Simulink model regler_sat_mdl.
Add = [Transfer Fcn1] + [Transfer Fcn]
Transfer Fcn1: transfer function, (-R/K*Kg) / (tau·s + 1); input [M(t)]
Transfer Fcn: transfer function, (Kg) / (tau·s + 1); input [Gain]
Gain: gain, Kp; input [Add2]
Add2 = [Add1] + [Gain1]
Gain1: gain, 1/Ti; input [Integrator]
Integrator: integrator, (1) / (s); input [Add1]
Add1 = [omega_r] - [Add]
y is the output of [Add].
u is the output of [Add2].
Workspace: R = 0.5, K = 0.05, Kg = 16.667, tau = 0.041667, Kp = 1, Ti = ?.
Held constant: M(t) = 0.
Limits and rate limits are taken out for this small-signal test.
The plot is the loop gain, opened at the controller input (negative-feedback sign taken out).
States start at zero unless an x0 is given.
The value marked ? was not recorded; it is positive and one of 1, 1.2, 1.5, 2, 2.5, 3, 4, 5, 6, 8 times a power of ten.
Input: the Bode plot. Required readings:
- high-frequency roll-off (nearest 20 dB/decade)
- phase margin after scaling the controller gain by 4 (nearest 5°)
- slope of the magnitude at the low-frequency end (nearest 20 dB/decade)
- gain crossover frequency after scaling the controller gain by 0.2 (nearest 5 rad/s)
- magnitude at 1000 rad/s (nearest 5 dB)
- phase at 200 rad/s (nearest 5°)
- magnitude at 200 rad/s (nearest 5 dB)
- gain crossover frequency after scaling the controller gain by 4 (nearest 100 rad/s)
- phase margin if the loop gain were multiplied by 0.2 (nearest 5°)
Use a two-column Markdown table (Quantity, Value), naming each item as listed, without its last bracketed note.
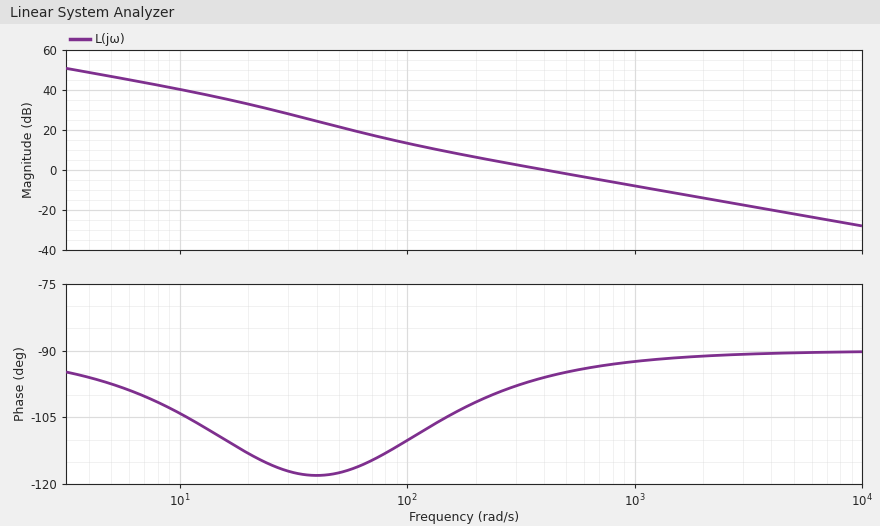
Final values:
| Quantity | Value |
|---|---|
| high-frequency roll-off | -20 dB/decade |
| phase margin after scaling the controller gain by 4 | 90° |
| slope of the magnitude at the low-frequency end | -20 dB/decade |
| gain crossover frequency after scaling the controller gain by 0.2 | 95 rad/s |
| magnitude at 1000 rad/s | -10 dB |
| phase at 200 rad/s | -100° |
| magnitude at 200 rad/s | 5 dB |
| gain crossover frequency after scaling the controller gain by 4 | 1600 rad/s |
| phase margin if the loop gain were multiplied by 0.2 | 70° |
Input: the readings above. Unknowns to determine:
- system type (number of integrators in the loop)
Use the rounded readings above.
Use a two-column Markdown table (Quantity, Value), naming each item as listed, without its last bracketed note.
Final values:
| Quantity | Value |
|---|---|
| system type | 1 |
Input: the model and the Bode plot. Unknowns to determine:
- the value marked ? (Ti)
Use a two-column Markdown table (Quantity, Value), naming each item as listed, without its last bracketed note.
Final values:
| Quantity | Value |
|---|---|
| the value marked ? | 0.015 |
